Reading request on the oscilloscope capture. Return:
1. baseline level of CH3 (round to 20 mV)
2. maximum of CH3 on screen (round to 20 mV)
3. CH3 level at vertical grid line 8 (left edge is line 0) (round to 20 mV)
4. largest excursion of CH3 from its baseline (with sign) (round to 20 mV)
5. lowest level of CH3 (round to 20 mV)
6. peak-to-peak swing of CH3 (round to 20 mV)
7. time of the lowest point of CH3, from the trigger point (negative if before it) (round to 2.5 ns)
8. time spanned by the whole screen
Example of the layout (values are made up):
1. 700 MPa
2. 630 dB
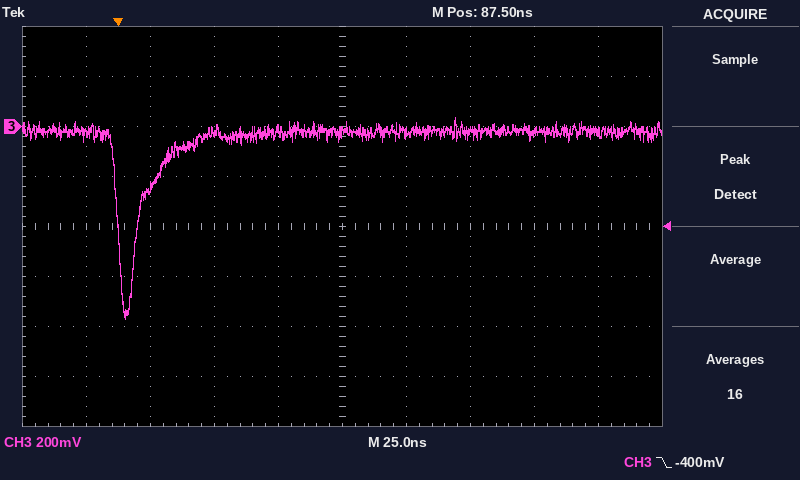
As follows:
1. -20 mV
2. 40 mV
3. -20 mV
4. -740 mV
5. -760 mV
6. 800 mV
7. +2.5 ns
8. 250 ns
